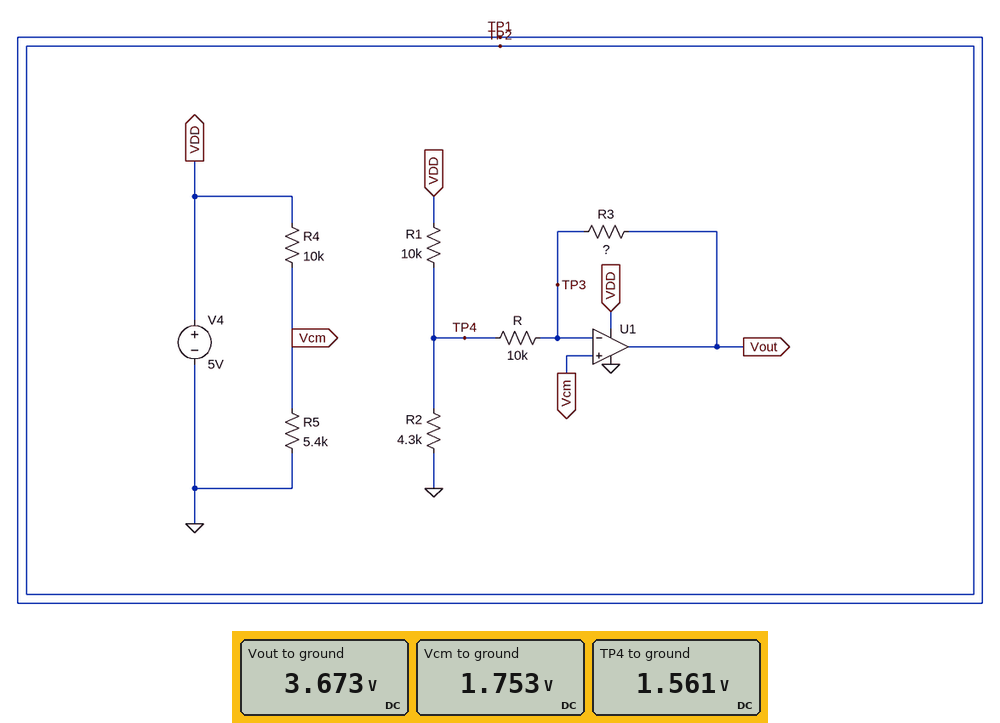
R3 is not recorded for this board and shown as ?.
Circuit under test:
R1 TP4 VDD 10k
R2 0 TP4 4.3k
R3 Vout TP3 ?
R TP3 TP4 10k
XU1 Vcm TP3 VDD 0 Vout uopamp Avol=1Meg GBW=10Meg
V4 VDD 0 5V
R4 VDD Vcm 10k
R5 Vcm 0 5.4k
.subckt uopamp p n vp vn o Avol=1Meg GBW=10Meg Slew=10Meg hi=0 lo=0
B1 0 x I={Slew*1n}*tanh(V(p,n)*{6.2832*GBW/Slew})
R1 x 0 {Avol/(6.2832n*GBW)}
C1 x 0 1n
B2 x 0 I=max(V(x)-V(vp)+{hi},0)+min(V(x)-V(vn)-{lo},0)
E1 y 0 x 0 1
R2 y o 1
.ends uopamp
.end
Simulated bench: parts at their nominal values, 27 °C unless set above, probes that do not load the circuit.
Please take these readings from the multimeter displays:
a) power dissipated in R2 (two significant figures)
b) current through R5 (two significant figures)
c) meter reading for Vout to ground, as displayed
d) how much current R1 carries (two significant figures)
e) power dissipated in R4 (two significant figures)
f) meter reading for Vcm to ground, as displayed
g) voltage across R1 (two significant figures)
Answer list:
570 µW
320 µA
3.673 V
340 µA
1.1 mW
1.753 V
3.4 V
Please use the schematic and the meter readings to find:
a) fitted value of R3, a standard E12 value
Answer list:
100 kΩ
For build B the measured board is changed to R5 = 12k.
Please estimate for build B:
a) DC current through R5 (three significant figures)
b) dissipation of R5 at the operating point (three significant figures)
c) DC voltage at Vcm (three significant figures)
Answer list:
227 µA
620 µW
2.73 V
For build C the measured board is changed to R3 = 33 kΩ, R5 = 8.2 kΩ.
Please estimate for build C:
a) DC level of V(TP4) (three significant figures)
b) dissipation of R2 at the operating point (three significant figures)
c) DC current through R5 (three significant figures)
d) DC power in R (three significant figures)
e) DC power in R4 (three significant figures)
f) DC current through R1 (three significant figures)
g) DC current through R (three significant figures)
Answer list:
1.68 V
654 µW
275 µA
33.2 µW
755 µW
332 µA
57.6 µA
